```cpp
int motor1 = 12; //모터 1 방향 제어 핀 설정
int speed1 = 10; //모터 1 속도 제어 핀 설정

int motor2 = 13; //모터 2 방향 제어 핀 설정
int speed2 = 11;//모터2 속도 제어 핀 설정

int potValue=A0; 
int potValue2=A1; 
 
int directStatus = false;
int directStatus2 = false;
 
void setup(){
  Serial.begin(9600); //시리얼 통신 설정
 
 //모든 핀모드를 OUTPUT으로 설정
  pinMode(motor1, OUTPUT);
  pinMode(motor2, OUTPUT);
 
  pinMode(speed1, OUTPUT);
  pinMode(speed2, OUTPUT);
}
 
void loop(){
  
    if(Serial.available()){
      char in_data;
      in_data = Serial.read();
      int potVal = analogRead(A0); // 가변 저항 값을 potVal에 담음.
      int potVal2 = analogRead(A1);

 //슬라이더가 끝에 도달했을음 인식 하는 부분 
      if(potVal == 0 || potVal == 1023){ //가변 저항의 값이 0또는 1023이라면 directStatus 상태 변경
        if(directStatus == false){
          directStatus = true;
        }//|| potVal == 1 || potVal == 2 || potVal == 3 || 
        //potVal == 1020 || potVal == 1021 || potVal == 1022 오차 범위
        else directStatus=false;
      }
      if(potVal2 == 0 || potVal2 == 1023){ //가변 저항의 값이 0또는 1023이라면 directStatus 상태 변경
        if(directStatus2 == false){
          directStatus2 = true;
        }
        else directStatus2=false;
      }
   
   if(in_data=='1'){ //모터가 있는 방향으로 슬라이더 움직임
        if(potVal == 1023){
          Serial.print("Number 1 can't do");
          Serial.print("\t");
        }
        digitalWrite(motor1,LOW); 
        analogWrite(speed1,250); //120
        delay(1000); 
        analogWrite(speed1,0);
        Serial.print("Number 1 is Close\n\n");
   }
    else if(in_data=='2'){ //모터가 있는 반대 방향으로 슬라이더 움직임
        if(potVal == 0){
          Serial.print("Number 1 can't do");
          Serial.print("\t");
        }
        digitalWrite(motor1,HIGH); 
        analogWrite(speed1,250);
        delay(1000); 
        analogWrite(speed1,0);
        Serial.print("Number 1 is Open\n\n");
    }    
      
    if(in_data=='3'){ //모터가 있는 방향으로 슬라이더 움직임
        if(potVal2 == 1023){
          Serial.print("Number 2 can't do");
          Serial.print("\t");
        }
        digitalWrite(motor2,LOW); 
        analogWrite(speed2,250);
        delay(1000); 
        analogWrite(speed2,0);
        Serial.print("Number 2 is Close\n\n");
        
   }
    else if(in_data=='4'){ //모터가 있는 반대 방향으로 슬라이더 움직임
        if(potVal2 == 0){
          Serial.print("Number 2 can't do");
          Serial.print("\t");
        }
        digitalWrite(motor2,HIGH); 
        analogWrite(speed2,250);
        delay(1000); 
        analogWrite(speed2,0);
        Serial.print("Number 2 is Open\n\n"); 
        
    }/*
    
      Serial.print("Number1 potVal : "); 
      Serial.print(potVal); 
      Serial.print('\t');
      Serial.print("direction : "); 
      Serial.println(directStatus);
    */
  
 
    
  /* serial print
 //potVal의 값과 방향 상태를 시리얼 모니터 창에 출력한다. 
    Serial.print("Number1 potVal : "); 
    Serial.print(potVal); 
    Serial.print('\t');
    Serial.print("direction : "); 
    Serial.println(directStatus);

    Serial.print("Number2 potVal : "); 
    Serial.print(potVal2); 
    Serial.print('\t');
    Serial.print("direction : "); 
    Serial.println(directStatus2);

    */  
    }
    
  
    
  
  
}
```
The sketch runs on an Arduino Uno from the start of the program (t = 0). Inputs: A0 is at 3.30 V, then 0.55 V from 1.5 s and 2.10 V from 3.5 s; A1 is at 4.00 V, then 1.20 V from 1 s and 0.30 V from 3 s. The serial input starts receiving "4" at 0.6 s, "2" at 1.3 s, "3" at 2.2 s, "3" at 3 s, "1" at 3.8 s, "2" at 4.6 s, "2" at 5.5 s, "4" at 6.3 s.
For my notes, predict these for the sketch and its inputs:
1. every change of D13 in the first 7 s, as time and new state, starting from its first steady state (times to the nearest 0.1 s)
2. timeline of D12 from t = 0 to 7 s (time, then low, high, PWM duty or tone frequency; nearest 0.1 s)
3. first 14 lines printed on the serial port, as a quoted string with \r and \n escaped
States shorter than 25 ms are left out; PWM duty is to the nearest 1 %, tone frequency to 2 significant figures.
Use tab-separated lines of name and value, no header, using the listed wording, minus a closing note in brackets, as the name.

every change of D13 in the first 7 s, as time and new state, starting from its first steady state	0 s low; 0.6 s high; 2.6 s low
timeline of D12 from t = 0 to 7 s	0 s low; 1.6 s high; 4.6 s low; 5.6 s high
first 14 lines printed on the serial port, as a quoted string with \r and \n escaped	"Number 2 is Open\n\nNumber 1 is Open\n\nNumber 2 is Close\n\nNumber 2 is Close\n\nNumber 1 is Close\n\nNumber 1 is Open\n\nNumber 1 is Open\n\n"
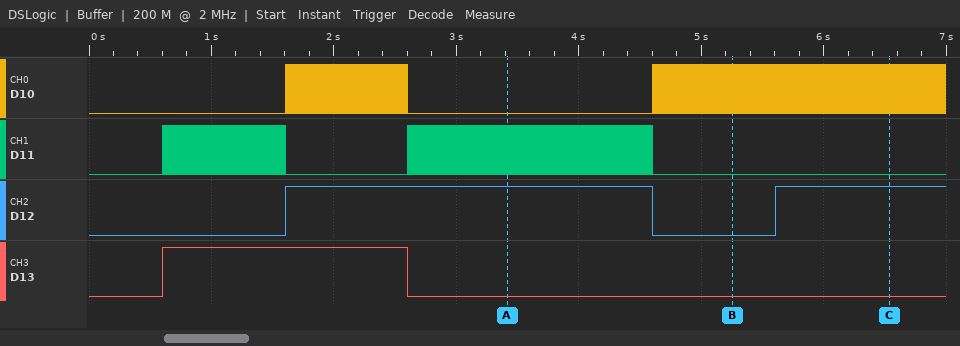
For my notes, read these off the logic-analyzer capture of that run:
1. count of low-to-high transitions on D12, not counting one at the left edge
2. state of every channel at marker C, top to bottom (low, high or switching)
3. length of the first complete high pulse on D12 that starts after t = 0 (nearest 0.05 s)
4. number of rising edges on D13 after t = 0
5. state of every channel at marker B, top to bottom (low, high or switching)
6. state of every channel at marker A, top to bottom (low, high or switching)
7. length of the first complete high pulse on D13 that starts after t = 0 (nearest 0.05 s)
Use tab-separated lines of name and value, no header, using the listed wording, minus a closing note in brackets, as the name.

count of low-to-high transitions on D12, not counting one at the left edge	2
state of every channel at marker C, top to bottom	D10 switching, D11 low, D12 high, D13 low
length of the first complete high pulse on D12 that starts after t = 0	3.00 s
number of rising edges on D13 after t = 0	1
state of every channel at marker B, top to bottom	D10 switching, D11 low, D12 low, D13 low
state of every channel at marker A, top to bottom	D10 low, D11 switching, D12 high, D13 low
length of the first complete high pulse on D13 that starts after t = 0	2.00 s
